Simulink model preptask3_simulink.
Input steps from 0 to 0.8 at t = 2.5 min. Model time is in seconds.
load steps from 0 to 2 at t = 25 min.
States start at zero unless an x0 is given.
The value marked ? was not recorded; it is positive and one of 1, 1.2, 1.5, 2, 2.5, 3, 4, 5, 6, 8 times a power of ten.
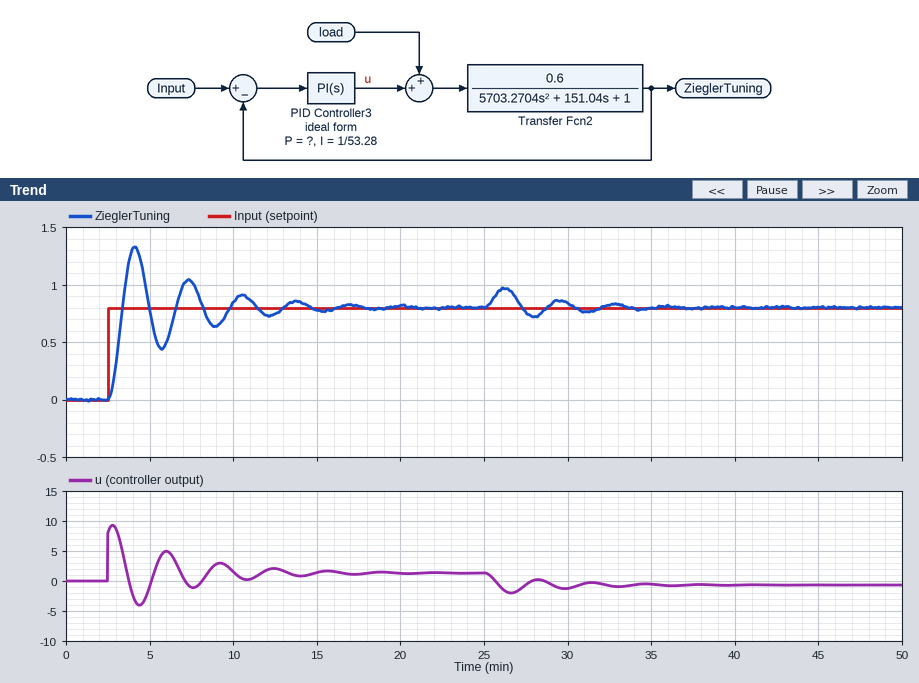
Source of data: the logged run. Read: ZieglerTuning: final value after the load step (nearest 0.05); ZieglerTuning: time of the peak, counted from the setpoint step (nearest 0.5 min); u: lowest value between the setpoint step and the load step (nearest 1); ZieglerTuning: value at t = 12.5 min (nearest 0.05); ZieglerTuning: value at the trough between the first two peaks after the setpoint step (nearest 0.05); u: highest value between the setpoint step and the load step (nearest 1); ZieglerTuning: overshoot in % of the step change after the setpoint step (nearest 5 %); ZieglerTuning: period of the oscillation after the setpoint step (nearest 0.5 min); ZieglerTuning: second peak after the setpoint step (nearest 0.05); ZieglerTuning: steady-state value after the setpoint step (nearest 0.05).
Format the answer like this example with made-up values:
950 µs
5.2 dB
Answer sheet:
0.80
1.5 min
-4
0.75
0.45
9
65 %
3.0 min
1.05
0.80
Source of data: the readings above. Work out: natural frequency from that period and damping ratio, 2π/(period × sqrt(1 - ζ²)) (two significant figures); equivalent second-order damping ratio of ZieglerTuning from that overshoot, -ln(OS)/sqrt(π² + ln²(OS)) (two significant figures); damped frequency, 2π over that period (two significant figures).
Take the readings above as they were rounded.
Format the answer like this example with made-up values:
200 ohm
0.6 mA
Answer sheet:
2.1 rad/min
0.14
2.1 rad/min
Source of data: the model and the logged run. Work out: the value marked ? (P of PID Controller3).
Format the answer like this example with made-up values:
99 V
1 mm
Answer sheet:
10
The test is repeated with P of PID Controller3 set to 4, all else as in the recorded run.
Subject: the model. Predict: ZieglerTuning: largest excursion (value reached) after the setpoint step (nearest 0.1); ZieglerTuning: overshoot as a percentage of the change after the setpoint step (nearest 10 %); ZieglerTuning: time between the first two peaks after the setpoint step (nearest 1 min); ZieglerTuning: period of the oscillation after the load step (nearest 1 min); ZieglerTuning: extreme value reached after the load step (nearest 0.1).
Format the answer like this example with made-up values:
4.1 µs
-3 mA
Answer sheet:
1.2
50 %
5 min
5 min
1.1
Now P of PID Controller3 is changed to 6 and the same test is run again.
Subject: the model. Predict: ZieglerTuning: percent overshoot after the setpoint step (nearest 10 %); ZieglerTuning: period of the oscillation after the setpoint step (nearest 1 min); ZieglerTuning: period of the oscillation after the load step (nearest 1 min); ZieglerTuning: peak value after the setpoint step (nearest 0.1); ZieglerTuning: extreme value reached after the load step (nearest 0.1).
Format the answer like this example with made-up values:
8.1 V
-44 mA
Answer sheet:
60 %
4 min
4 min
1.3
1.0
